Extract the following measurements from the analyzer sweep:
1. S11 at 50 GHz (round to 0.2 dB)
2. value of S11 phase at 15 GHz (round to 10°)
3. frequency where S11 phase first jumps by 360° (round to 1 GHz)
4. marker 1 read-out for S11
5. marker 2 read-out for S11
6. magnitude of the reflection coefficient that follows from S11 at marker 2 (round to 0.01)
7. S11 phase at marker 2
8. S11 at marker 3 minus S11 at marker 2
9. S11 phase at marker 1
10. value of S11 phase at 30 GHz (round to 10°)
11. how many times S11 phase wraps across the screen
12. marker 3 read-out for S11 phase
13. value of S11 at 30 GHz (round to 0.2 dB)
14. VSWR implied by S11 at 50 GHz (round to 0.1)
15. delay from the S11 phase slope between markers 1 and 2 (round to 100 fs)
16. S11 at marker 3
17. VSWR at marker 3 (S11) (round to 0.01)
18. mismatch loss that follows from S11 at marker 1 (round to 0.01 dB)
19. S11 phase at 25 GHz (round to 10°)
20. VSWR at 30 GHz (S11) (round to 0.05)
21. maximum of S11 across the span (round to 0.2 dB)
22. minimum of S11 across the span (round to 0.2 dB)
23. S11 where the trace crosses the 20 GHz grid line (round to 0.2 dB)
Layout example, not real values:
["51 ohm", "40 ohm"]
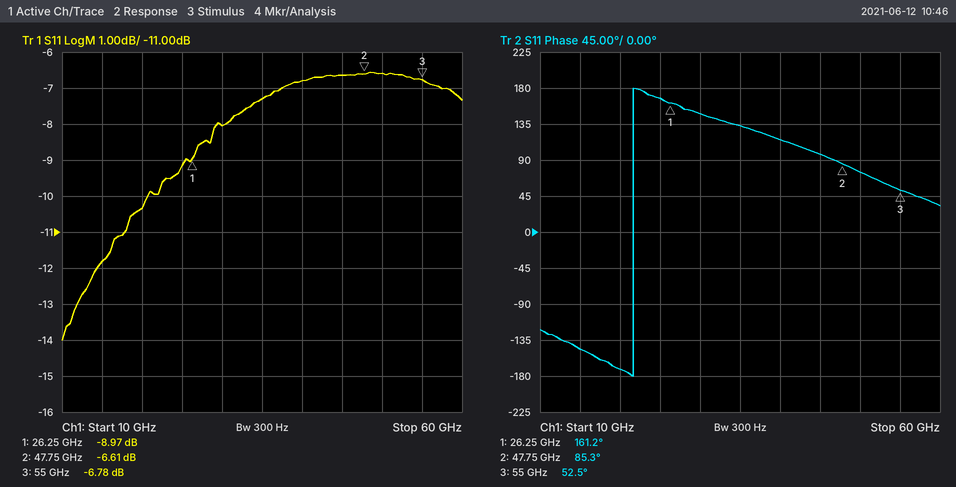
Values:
["-6.6 dB", "-150°", "22 GHz", "-8.97 dB", "-6.61 dB", "0.47", "85.3°", "-0.17 dB", "161.2°", "150°", "1", "52.5°", "-8.0 dB", "2.8", "9.8 ps", "-6.78 dB", "2.69", "0.59 dB", "170°", "2.30", "-6.6 dB", "-14.0 dB", "-10.4 dB"]
